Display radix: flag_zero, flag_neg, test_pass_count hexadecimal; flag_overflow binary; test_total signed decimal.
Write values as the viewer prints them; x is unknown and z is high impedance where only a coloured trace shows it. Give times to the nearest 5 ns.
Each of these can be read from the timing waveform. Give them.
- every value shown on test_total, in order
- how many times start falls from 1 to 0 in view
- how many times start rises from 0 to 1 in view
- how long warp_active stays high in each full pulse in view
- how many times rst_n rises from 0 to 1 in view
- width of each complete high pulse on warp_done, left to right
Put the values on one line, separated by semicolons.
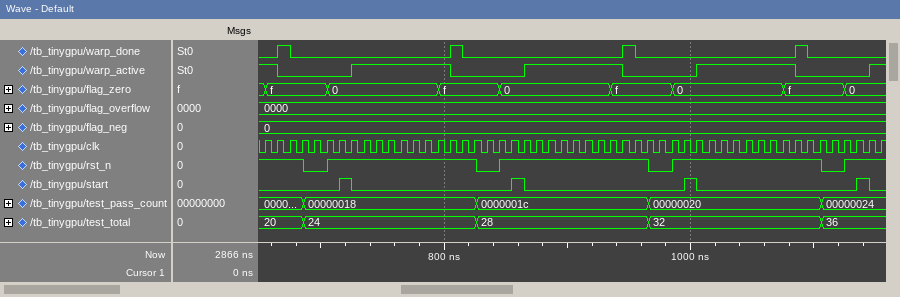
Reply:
20, 24, 28, 32, 36; 4; 4; 80 ns, 80 ns, 80 ns; 4; 10 ns, 10 ns, 10 ns, 10 ns
